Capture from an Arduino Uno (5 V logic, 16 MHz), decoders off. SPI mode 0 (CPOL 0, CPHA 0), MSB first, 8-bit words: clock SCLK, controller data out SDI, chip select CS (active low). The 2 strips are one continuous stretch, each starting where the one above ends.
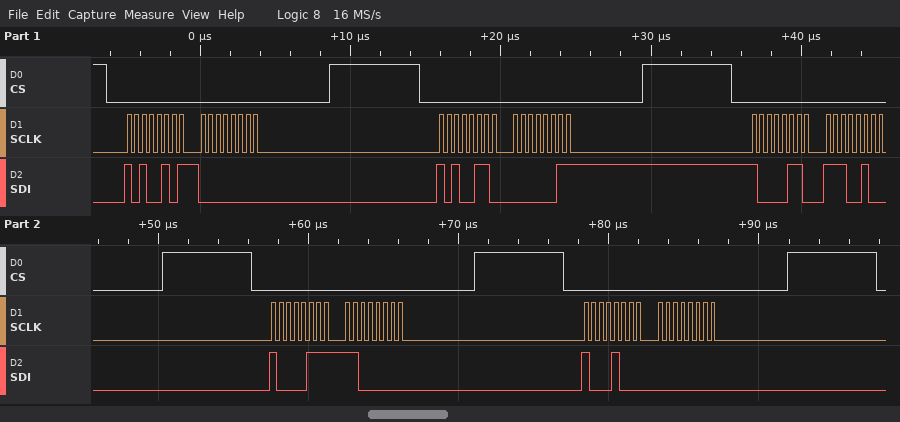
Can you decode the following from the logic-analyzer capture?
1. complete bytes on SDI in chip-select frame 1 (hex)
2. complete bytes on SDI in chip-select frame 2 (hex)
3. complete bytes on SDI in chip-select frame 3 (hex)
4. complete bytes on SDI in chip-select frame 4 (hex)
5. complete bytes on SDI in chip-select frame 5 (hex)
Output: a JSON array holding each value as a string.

["0xA5 0x00", "0xA6 0x03", "0x86 0xE4", "0x87 0xC0", "0x88 0x00"]
